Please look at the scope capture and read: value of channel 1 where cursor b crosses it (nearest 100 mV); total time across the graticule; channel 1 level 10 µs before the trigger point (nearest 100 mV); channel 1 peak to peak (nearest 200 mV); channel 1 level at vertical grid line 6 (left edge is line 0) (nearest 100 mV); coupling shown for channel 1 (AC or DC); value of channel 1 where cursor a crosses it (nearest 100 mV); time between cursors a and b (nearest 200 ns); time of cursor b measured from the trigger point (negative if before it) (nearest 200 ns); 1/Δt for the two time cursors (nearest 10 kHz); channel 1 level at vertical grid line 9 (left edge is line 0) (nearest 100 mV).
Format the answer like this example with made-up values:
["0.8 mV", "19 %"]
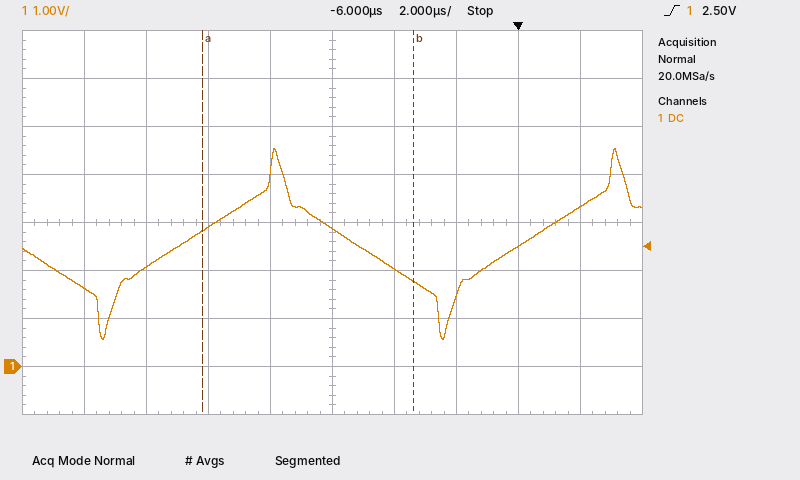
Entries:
["1.8 V", "20 µs", "2.9 V", "4.0 V", "2.0 V", "DC", "2.8 V", "6.8 µs", "-3.4 µs", "150 kHz", "3.3 V"]
